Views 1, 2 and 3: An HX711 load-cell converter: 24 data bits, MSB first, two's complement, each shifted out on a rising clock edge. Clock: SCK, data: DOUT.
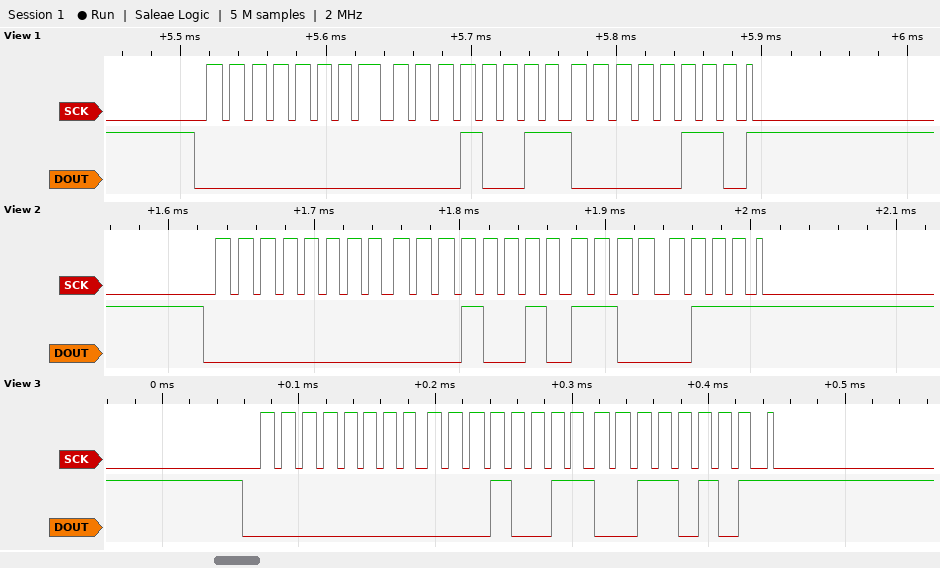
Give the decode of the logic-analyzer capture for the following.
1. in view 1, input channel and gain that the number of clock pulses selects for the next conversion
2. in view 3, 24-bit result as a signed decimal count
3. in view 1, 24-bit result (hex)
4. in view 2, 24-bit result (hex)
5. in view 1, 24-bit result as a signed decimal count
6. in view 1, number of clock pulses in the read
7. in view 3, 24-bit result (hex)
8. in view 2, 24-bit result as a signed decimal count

channel A, gain 128
4917
0x001306
0x0012C7
4870
25
0x001335
4807
